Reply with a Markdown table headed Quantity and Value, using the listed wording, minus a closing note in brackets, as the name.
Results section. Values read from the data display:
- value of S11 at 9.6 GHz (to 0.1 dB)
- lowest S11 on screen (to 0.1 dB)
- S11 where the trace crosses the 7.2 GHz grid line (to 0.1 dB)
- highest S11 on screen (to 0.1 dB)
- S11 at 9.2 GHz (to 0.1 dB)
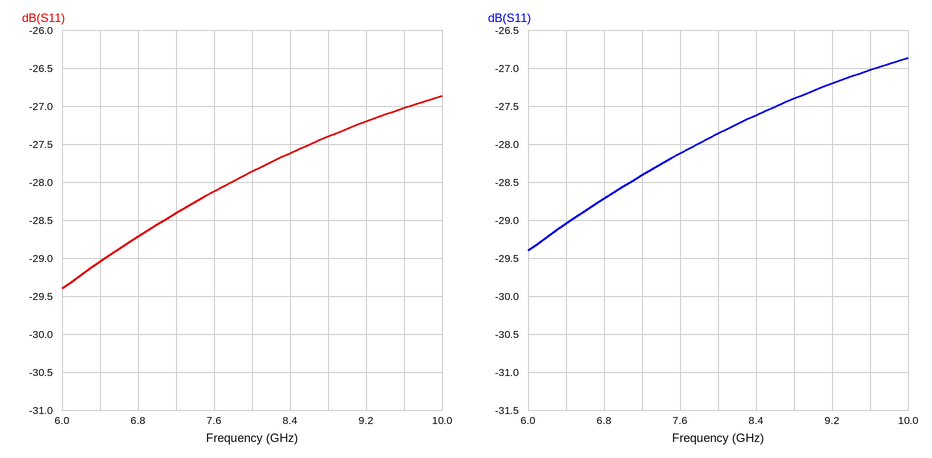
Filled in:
| Quantity | Value |
|---|---|
| value of S11 at 9.6 GHz | -27.0 dB |
| lowest S11 on screen | -29.4 dB |
| S11 where the trace crosses the 7.2 GHz grid line | -28.4 dB |
| highest S11 on screen | -26.9 dB |
| S11 at 9.2 GHz | -27.2 dB |
